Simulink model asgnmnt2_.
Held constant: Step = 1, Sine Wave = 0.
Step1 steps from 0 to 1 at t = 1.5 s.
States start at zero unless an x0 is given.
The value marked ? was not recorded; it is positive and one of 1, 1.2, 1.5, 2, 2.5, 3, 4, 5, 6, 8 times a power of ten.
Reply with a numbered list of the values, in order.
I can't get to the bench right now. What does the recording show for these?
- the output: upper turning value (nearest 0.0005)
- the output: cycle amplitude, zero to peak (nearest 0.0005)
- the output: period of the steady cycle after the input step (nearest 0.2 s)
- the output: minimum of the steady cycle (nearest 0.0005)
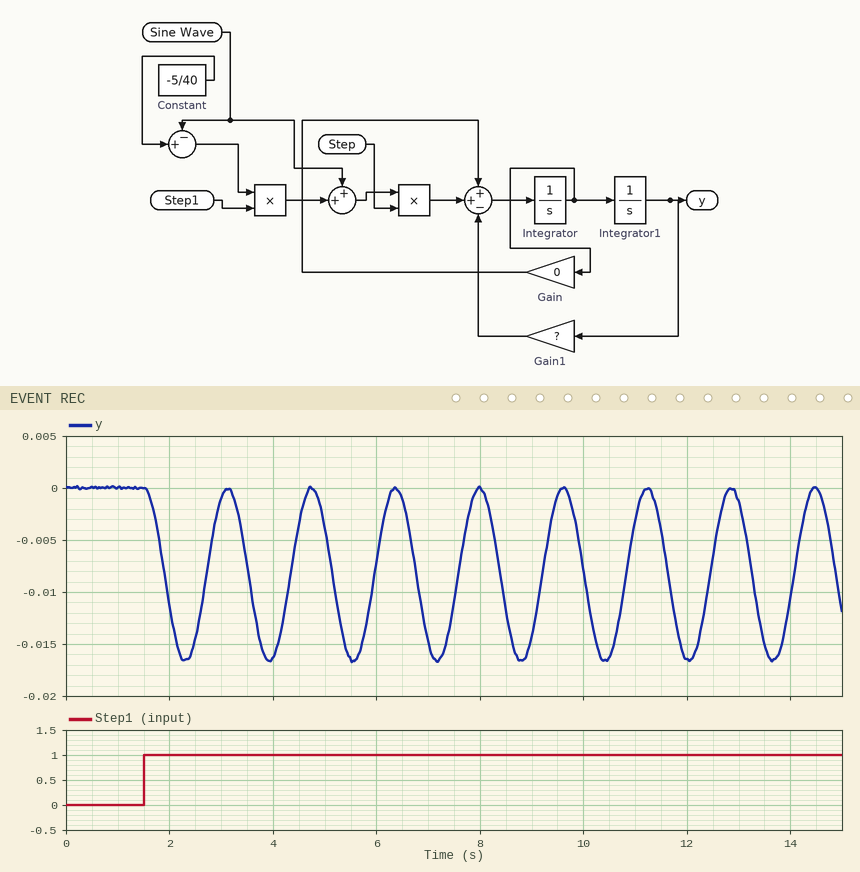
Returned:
1. 0.0000
2. 0.0085
3. 1.6 s
4. -0.0165
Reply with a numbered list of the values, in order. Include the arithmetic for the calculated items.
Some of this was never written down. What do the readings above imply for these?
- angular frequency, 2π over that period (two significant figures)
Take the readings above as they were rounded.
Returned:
1. 2π / 1.6 = 3.9 rad/s
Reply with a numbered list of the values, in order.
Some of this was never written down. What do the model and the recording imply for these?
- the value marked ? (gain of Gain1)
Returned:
1. 15
